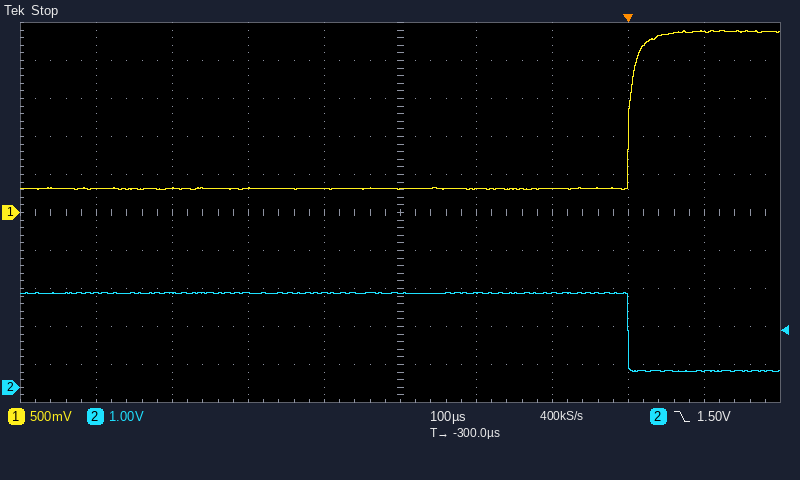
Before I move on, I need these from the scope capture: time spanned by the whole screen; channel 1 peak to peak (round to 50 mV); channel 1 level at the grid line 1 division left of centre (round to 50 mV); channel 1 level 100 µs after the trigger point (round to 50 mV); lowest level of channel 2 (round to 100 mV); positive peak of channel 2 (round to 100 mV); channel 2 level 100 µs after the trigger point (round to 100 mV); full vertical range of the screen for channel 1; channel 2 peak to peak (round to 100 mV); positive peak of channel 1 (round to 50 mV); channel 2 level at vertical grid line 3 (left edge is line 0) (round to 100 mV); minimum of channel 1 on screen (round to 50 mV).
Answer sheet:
1 ms
2.10 V
300 mV
2.40 V
400 mV
2.5 V
400 mV
5 V
2.1 V
2.40 V
2.5 V
300 mV
